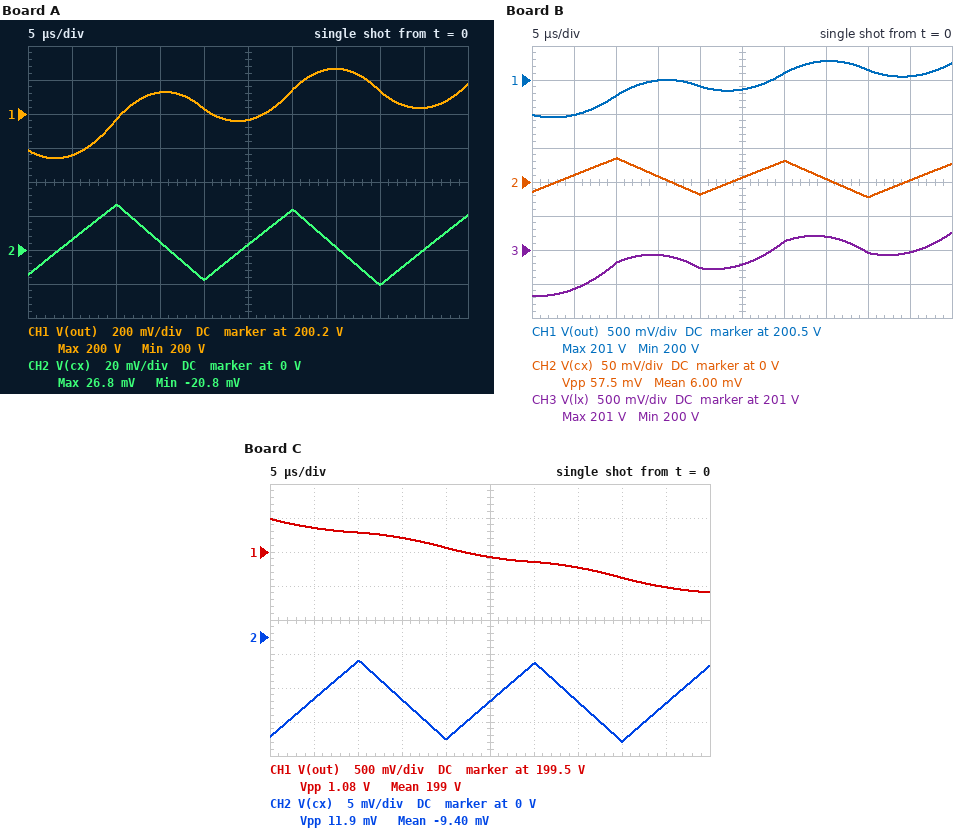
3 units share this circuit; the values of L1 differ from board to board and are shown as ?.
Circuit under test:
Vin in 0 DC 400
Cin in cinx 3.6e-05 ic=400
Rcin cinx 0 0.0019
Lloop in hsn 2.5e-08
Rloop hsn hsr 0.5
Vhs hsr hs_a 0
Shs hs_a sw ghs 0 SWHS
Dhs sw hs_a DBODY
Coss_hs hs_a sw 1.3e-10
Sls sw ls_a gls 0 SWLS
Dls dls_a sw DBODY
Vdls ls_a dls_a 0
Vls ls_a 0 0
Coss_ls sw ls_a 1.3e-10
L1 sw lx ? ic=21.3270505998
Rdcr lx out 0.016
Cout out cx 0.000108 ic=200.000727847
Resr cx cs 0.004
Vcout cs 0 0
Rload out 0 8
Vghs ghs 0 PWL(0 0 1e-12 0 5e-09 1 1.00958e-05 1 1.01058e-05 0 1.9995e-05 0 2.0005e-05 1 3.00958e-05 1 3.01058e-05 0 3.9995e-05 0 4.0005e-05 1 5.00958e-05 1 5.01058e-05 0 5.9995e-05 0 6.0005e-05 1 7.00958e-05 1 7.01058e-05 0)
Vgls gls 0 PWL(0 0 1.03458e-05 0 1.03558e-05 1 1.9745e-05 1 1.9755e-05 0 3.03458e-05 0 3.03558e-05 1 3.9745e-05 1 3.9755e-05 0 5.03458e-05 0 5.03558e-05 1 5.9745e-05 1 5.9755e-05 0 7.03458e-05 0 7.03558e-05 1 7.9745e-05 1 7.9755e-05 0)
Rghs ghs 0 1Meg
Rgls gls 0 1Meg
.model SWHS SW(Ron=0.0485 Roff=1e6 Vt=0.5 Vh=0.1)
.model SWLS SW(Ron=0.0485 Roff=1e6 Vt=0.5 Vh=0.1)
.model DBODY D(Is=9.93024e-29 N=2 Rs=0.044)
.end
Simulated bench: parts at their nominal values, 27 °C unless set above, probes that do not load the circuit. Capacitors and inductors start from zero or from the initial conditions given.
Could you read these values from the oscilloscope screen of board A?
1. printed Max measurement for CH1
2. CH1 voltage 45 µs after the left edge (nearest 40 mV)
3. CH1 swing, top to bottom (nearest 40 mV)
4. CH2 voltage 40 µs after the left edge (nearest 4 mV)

200 V
200.24 V
520 mV
-20 mV
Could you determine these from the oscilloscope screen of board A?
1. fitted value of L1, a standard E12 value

180 µH
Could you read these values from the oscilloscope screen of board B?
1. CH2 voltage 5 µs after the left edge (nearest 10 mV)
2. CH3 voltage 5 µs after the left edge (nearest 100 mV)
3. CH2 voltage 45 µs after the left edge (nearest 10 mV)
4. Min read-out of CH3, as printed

10 mV
200.4 V
0 V
200 V
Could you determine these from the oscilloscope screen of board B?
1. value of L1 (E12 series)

150 µH
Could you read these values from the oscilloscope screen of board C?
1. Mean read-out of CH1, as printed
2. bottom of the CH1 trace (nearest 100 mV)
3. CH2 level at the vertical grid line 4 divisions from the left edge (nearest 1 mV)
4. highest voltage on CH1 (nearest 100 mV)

199 V
198.9 V
-15 mV
200.0 V
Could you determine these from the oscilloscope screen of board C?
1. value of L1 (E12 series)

680 µH
